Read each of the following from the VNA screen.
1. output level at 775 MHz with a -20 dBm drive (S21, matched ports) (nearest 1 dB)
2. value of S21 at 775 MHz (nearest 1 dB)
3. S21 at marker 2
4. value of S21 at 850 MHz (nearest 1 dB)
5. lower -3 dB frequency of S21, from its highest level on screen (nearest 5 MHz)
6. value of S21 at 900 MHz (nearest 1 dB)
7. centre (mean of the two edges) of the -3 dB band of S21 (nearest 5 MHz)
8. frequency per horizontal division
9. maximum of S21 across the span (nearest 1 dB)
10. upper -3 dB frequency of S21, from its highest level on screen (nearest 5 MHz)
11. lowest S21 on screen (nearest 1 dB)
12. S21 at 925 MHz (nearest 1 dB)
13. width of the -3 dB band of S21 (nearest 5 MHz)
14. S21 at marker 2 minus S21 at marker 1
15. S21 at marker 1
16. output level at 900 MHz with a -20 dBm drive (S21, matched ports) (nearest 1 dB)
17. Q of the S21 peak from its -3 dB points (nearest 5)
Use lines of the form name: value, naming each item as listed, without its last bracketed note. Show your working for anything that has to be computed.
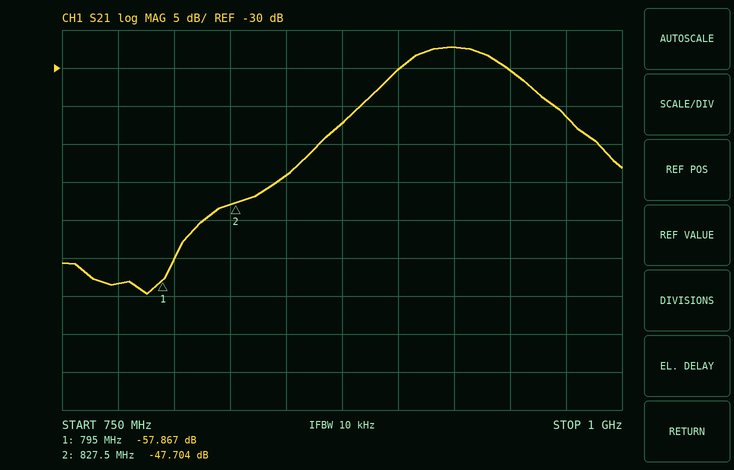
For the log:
output level at 775 MHz with a -20 dBm drive (S21, matched ports): -20 dBm + (-58 dB) = -78 dBm
value of S21 at 775 MHz: -58 dB
S21 at marker 2: -47.704 dB
value of S21 at 850 MHz: -44 dB
lower -3 dB frequency of S21, from its highest level on screen: 900 MHz
value of S21 at 900 MHz: -30 dB
centre (mean of the two edges) of the -3 dB band of S21: 925 MHz
frequency per horizontal division: 25 MHz
maximum of S21 across the span: -27 dB
upper -3 dB frequency of S21, from its highest level on screen: 950 MHz
lowest S21 on screen: -60 dB
S21 at 925 MHz: -27 dB
width of the -3 dB band of S21: 950 MHz − 900 MHz = 50 MHz
S21 at marker 2 minus S21 at marker 1: -47.704 − (-57.867) = 10.163 dB
S21 at marker 1: -57.867 dB
output level at 900 MHz with a -20 dBm drive (S21, matched ports): -20 dBm + (-30 dB) = -50 dBm
Q of the S21 peak from its -3 dB points: 925 MHz / 50 MHz ≈ 18.5, so 20 to the nearest 5
